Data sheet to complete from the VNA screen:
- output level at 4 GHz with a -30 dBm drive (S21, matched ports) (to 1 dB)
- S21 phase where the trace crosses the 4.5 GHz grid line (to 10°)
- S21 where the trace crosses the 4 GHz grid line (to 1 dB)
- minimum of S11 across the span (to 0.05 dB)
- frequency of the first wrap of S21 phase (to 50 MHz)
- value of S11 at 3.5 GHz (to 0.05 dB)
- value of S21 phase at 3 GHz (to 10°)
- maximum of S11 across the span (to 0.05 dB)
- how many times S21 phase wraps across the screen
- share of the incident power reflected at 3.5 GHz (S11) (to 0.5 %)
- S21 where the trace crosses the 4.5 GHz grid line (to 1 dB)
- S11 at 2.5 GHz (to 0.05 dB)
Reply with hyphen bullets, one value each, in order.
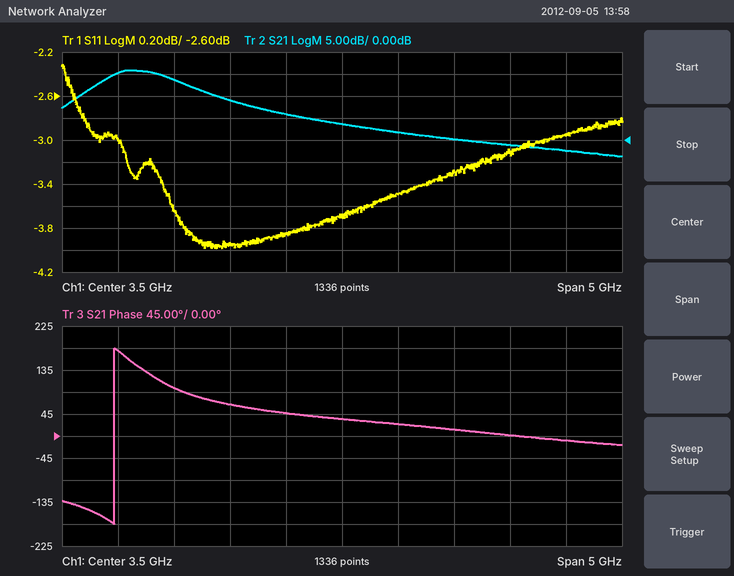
- -28 dBm
- 10°
- 2 dB
- -4.00 dB
- 1.45 GHz
- -3.70 dB
- 50°
- -2.30 dB
- 1
- 42.5 %
- 0 dB
- -3.95 dB
